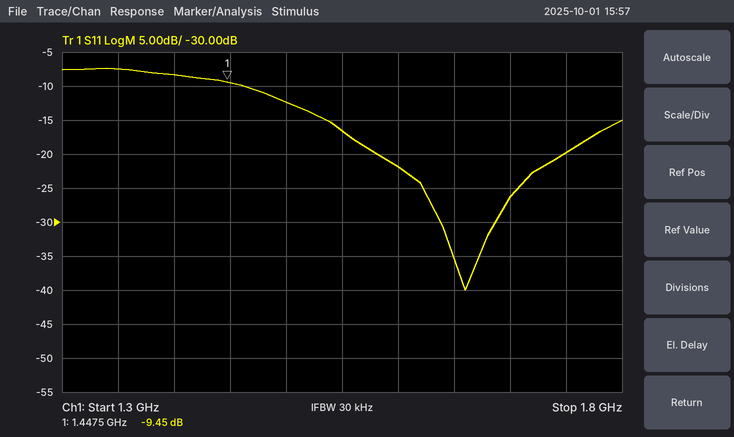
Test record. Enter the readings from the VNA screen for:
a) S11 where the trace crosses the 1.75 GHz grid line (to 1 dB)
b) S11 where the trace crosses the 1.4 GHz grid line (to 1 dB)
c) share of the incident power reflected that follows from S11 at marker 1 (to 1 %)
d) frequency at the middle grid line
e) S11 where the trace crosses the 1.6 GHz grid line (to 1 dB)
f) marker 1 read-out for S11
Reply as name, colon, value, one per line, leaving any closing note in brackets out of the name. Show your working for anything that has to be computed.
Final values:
S11 where the trace crosses the 1.75 GHz grid line: -20 dB
S11 where the trace crosses the 1.4 GHz grid line: -8 dB
share of the incident power reflected that follows from S11 at marker 1: 10^(-9.45/10) ≈ 11 %
frequency at the middle grid line: 1.55 GHz
S11 where the trace crosses the 1.6 GHz grid line: -22 dB
marker 1 read-out for S11: -9.45 dB
